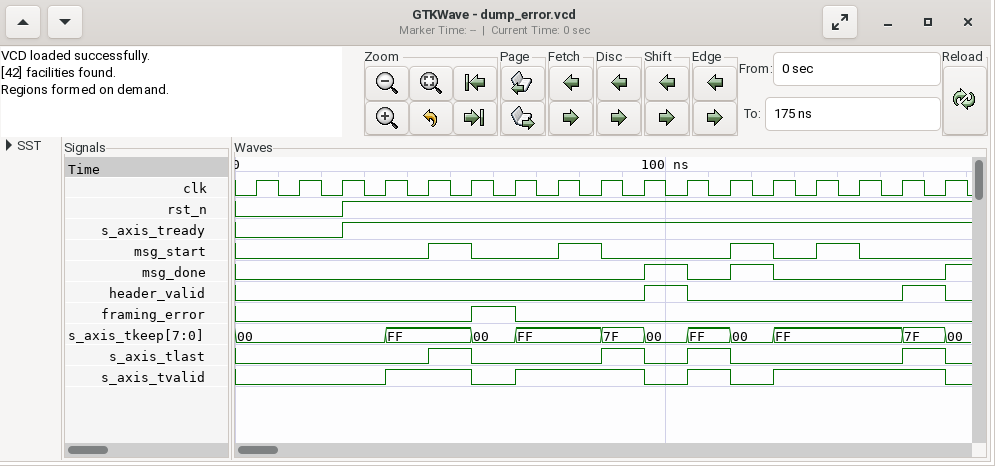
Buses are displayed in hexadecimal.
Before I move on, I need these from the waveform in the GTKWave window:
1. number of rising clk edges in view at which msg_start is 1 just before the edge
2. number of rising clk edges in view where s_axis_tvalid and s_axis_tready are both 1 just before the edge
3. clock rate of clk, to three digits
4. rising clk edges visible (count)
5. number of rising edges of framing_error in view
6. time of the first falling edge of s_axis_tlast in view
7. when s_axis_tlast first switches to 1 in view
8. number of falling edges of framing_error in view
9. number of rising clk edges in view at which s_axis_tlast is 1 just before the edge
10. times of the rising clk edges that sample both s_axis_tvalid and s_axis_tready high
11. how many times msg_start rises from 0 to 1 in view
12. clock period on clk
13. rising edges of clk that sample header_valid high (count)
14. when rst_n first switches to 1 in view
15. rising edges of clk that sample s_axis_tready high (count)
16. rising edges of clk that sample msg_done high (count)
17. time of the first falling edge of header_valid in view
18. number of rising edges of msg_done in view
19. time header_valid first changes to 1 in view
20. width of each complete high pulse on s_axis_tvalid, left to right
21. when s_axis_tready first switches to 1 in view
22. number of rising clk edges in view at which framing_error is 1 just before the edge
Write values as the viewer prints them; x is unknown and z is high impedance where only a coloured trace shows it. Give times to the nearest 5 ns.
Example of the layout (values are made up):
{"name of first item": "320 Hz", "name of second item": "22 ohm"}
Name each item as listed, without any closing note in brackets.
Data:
{"number of rising clk edges in view at which msg_start is 1 just before the edge": "4", "number of rising clk edges in view where s_axis_tvalid and s_axis_tready are both 1 just before the edge": "10", "clock rate of clk, to three digits": "100 MHz", "rising clk edges visible": "17", "number of rising edges of framing_error in view": "1", "time of the first falling edge of s_axis_tlast in view": "55 ns", "when s_axis_tlast first switches to 1 in view": "45 ns", "number of falling edges of framing_error in view": "1", "number of rising clk edges in view at which s_axis_tlast is 1 just before the edge": "4", "times of the rising clk edges that sample both s_axis_tvalid and s_axis_tready high": "45 ns, 55 ns, 75 ns, 85 ns, 95 ns, 115 ns, 135 ns, 145 ns, 155 ns, 165 ns", "how many times msg_start rises from 0 to 1 in view": "4", "clock period on clk": "10 ns", "rising edges of clk that sample header_valid high": "2", "when rst_n first switches to 1 in view": "25 ns", "rising edges of clk that sample s_axis_tready high": "14", "rising edges of clk that sample msg_done high": "2", "time of the first falling edge of header_valid in view": "105 ns", "number of rising edges of msg_done in view": "3", "time header_valid first changes to 1 in view": "95 ns", "width of each complete high pulse on s_axis_tvalid, left to right": "20 ns, 30 ns, 10 ns, 40 ns", "when s_axis_tready first switches to 1 in view": "25 ns", "number of rising clk edges in view at which framing_error is 1 just before the edge": "1"}
